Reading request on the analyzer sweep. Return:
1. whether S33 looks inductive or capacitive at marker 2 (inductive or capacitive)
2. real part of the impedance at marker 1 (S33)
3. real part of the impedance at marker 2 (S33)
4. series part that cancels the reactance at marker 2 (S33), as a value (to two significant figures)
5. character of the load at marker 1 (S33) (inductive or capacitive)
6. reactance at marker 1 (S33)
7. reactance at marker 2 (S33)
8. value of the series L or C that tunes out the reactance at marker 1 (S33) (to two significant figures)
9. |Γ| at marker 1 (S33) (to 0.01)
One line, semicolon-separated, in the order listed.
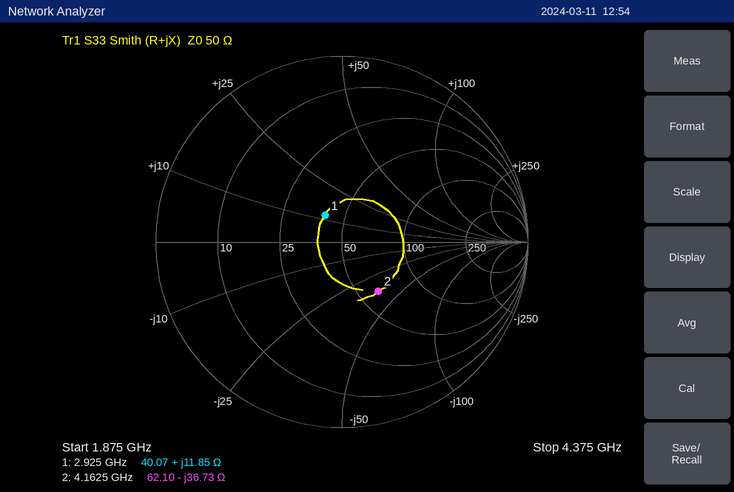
capacitive; 40.07 Ω; 62.10 Ω; 1.4 nH; inductive; +11.85 Ω; -36.73 Ω; 4.6 pF; 0.17
